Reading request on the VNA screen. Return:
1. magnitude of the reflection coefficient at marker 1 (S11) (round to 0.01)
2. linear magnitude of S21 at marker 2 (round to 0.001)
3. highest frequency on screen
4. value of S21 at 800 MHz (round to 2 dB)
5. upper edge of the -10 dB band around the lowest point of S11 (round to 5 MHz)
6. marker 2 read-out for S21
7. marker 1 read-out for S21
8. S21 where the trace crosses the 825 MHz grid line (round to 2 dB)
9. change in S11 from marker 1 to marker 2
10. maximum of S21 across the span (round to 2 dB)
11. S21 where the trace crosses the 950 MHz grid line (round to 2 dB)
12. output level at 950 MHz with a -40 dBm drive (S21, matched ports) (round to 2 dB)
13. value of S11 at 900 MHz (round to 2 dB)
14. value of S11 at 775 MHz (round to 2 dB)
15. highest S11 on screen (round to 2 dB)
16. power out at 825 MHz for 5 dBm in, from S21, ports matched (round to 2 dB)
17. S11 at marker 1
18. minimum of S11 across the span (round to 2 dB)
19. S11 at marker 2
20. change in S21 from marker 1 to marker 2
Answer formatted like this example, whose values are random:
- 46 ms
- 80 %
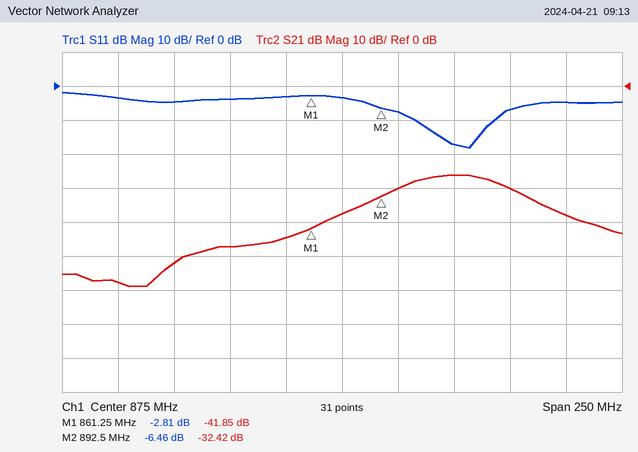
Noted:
- 0.72
- 0.024
- 1 GHz
- -52 dB
- 945 MHz
- -32.42 dB
- -41.85 dB
- -48 dB
- -3.65 dB
- -26 dB
- -30 dB
- -70 dBm
- -8 dB
- -4 dB
- -2 dB
- -42 dBm
- -2.81 dB
- -18 dB
- -6.46 dB
- 9.43 dB
